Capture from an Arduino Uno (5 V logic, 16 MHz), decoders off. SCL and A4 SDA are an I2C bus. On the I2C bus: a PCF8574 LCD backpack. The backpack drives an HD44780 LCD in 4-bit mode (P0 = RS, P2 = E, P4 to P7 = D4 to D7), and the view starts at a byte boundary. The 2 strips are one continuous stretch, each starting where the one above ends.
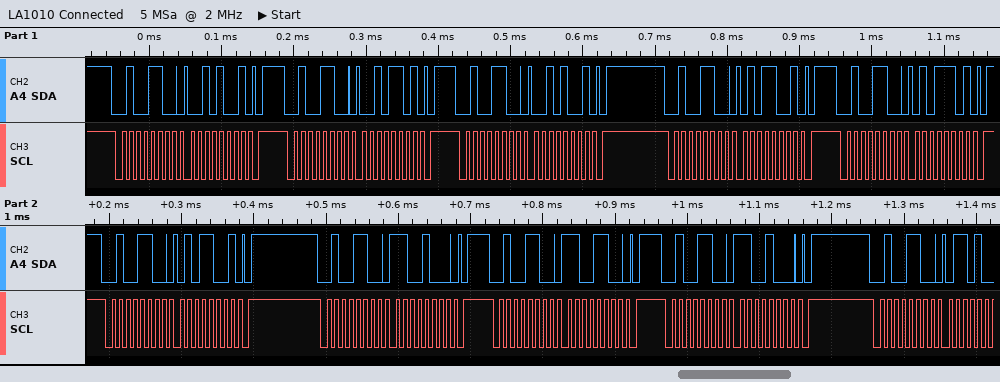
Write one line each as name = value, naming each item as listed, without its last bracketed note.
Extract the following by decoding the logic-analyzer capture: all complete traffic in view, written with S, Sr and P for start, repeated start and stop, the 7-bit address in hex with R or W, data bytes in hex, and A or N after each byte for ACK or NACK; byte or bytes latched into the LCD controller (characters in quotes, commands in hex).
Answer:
all complete traffic in view, written with S, Sr and P for start, repeated start and stop, the 7-bit address in hex with R or W, data bytes in hex, and A or N after each byte for ACK or NACK = S 26W A 29 A P S 26W A 2D A P S 26W A 29 A P S 26W A 59 A P S 26W A 5D A P S 26W A 59 A P S 26W A C8 A P S 26W A CC A P S 26W A C8 A P S 26W A
byte or bytes latched into the LCD controller = '%'
